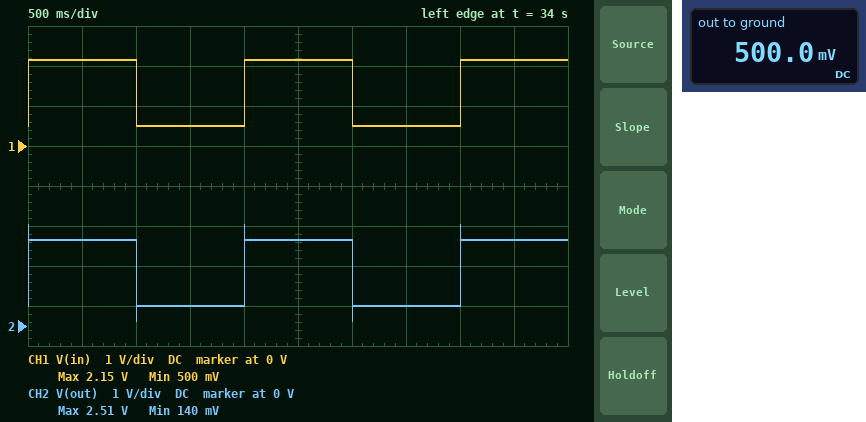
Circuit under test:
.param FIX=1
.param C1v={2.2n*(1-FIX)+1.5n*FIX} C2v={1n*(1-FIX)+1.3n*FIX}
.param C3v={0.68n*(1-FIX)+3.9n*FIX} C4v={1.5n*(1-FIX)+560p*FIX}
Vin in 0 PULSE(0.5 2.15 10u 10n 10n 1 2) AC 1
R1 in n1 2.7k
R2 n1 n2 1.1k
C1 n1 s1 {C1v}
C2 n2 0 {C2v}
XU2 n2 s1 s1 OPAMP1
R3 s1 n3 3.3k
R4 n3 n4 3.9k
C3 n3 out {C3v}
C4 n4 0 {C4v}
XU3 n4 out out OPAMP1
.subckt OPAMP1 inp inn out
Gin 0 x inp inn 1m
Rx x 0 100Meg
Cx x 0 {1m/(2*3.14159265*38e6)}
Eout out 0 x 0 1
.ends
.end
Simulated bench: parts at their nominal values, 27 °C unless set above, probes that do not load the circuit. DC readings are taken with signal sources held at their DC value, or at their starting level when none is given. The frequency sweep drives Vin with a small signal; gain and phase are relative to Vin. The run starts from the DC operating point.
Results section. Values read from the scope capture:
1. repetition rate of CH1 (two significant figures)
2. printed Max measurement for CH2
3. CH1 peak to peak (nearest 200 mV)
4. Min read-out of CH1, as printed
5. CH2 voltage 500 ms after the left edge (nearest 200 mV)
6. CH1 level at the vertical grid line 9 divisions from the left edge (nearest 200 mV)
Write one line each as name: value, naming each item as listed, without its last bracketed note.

repetition rate of CH1: 500 mHz
printed Max measurement for CH2: 2.51 V
CH1 peak to peak: 1.6 V
Min read-out of CH1, as printed: 500 mV
CH2 voltage 500 ms after the left edge: 2.2 V
CH1 level at the vertical grid line 9 divisions from the left edge: 2.2 V
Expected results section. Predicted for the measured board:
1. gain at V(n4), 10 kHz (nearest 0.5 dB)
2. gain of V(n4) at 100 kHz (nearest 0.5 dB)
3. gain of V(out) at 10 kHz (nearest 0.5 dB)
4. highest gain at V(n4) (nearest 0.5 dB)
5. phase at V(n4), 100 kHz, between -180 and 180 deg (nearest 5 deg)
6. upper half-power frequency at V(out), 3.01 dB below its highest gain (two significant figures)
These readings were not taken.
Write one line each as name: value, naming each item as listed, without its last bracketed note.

gain at V(n4), 10 kHz: 0.5 dB
gain of V(n4) at 100 kHz: -31.0 dB
gain of V(out) at 10 kHz: 0.5 dB
highest gain at V(n4): 2.0 dB
phase at V(n4), 100 kHz, between -180 and 180 deg: 80 deg
upper half-power frequency at V(out), 3.01 dB below its highest gain: 34 kHz
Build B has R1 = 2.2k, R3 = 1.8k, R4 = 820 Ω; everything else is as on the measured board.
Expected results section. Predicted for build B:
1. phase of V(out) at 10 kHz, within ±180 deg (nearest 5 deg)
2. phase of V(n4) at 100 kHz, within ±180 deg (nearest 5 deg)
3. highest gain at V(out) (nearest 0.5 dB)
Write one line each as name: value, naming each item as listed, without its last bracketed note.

phase of V(out) at 10 kHz, within ±180 deg: -20 deg
phase of V(n4) at 100 kHz, within ±180 deg: 145 deg
highest gain at V(out): 0 dB
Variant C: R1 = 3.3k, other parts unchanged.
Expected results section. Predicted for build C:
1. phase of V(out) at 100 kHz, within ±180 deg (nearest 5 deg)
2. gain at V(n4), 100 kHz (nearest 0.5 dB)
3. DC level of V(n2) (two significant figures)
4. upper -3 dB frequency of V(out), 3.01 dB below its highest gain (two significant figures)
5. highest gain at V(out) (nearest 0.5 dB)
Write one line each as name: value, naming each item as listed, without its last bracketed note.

phase of V(out) at 100 kHz, within ±180 deg: 75 deg
gain at V(n4), 100 kHz: -32.5 dB
DC level of V(n2): 500 mV
upper -3 dB frequency of V(out), 3.01 dB below its highest gain: 33 kHz
highest gain at V(out): 1.5 dB
